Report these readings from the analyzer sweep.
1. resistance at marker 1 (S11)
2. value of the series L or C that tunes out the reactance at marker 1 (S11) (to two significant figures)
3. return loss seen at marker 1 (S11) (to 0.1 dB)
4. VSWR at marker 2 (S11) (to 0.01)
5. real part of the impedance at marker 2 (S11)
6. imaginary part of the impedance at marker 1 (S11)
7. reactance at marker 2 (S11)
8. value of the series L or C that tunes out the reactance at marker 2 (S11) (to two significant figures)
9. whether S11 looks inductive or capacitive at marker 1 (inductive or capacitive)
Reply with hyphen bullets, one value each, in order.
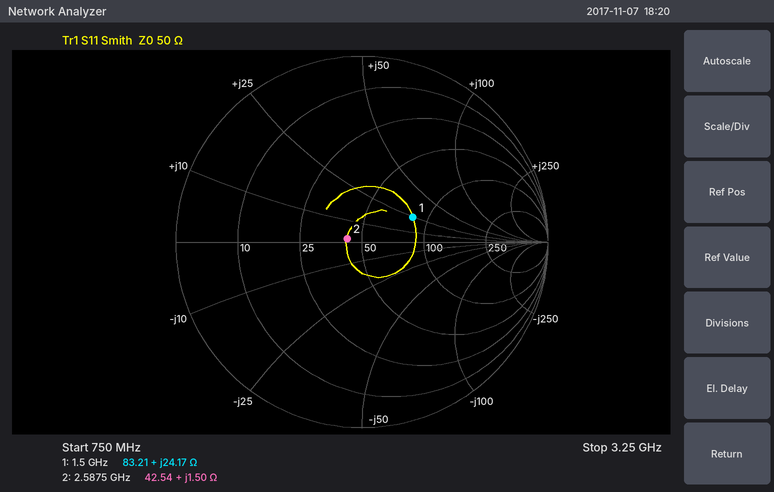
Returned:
- 83.21 Ω
- 4.4 pF
- 10.4 dB
- 1.18
- 42.54 Ω
- +24.17 Ω
- +1.50 Ω
- 41 pF
- inductive
